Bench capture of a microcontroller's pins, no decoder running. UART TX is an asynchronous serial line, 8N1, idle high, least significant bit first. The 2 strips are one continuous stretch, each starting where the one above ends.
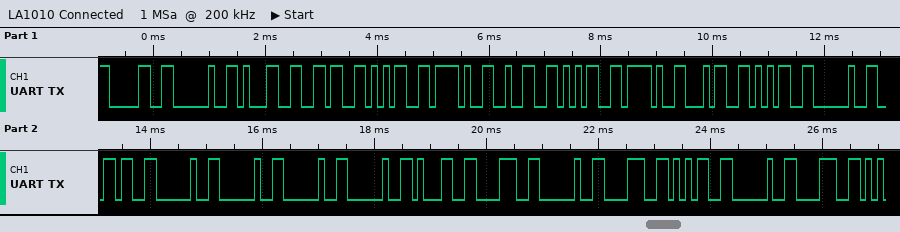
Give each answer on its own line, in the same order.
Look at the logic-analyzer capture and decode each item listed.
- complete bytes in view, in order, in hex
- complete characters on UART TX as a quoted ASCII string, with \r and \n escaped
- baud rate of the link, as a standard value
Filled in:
30 20 31 36 35 2F 32 35 2F 34 35 20 36 20 20 20 20 31 38 20 38 35 20 38
"0 165/25/45 6    18 85 8"
9600 baud
